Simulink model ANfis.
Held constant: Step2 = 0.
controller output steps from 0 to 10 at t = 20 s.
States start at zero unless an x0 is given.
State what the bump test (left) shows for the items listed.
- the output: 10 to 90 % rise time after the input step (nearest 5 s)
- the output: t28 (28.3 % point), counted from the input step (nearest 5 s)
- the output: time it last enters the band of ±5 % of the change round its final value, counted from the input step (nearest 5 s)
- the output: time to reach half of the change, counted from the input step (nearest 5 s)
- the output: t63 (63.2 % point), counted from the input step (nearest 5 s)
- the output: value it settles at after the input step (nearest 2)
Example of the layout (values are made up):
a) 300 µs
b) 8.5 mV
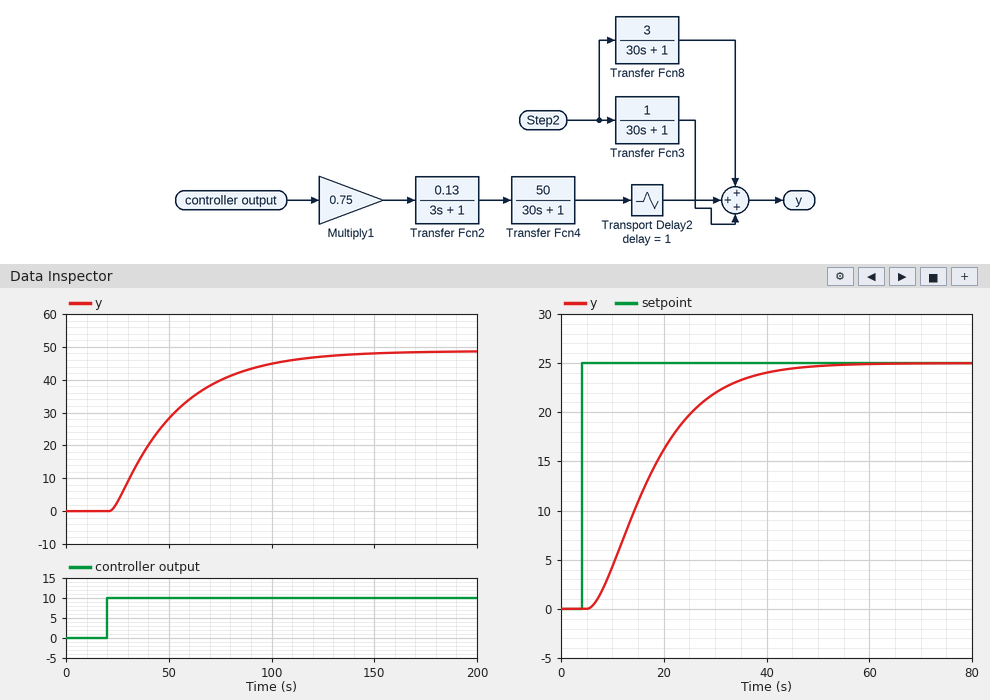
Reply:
a) 65 s
b) 15 s
c) 95 s
d) 25 s
e) 35 s
f) 48
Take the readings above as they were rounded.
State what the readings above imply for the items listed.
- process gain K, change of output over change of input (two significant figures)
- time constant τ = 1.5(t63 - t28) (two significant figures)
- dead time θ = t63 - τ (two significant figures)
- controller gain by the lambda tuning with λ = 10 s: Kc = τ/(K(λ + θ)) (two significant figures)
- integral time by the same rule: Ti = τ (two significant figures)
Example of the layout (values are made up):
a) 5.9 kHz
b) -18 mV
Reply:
a) 4.8
b) 30 s
c) 5.0 s
d) 0.42
e) 30 s
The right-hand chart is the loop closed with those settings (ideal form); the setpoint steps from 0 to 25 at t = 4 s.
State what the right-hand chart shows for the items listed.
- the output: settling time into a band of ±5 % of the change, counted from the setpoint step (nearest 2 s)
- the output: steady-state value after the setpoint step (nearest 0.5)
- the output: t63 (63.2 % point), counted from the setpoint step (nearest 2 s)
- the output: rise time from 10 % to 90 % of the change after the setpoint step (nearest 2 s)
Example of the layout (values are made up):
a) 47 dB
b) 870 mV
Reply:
a) 34 s
b) 25.0
c) 16 s
d) 24 s
